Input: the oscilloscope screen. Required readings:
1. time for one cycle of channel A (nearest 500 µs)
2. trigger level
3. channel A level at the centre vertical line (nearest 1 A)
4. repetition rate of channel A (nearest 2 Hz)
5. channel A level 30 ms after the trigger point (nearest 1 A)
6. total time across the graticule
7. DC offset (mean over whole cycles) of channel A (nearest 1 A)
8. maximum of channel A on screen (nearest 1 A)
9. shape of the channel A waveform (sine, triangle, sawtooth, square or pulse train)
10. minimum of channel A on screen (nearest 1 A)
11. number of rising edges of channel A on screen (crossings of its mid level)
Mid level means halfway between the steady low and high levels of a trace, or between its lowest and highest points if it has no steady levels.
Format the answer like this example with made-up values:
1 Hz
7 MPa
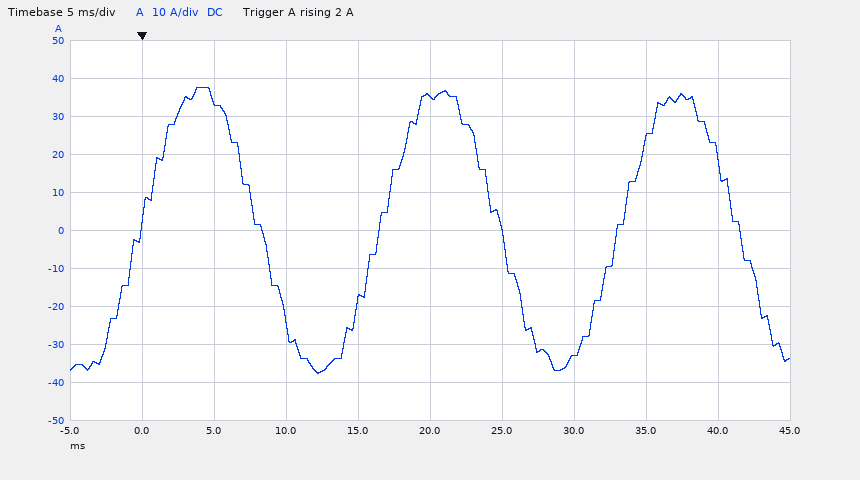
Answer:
16.5 ms
2 A
35 A
60 Hz
-33 A
50 ms
0 A
38 A
sine
-38 A
3
